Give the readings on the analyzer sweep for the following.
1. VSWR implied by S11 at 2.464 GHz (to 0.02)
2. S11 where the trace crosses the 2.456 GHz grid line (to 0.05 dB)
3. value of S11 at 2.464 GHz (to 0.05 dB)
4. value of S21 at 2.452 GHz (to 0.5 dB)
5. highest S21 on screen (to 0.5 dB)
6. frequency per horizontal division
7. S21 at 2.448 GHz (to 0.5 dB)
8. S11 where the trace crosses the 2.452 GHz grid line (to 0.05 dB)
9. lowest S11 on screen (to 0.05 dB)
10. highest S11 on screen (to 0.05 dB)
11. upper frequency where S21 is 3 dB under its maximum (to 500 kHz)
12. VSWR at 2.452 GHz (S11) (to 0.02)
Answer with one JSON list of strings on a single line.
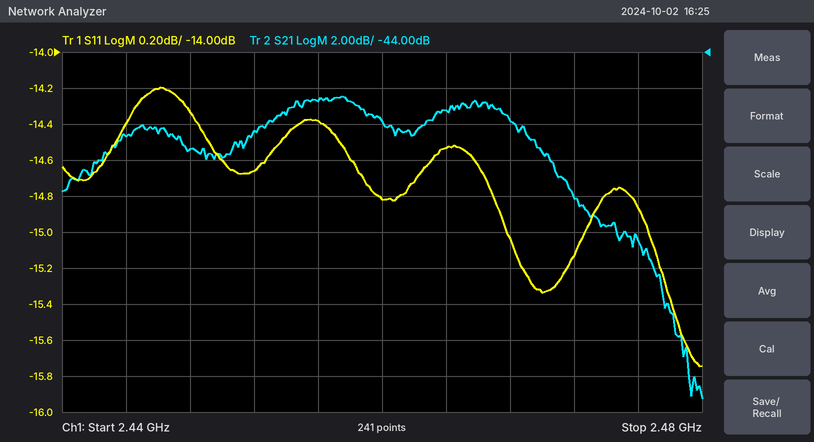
["1.46", "-14.40 dB", "-14.55 dB", "-48.5 dB", "-46.5 dB", "4 MHz", "-49.5 dB", "-14.65 dB", "-15.75 dB", "-14.20 dB", "2.4700 GHz", "1.46"]
